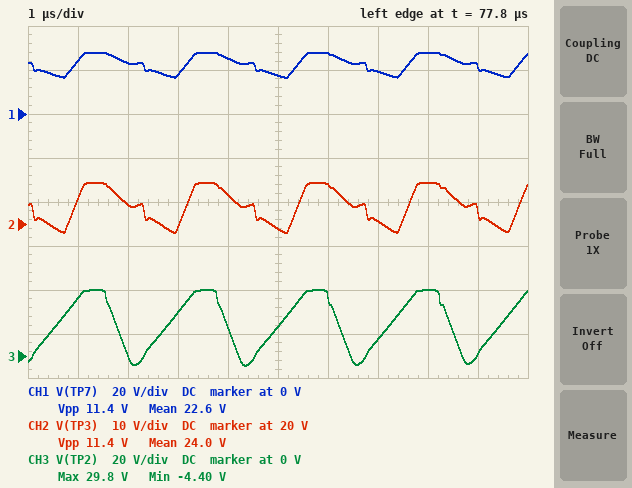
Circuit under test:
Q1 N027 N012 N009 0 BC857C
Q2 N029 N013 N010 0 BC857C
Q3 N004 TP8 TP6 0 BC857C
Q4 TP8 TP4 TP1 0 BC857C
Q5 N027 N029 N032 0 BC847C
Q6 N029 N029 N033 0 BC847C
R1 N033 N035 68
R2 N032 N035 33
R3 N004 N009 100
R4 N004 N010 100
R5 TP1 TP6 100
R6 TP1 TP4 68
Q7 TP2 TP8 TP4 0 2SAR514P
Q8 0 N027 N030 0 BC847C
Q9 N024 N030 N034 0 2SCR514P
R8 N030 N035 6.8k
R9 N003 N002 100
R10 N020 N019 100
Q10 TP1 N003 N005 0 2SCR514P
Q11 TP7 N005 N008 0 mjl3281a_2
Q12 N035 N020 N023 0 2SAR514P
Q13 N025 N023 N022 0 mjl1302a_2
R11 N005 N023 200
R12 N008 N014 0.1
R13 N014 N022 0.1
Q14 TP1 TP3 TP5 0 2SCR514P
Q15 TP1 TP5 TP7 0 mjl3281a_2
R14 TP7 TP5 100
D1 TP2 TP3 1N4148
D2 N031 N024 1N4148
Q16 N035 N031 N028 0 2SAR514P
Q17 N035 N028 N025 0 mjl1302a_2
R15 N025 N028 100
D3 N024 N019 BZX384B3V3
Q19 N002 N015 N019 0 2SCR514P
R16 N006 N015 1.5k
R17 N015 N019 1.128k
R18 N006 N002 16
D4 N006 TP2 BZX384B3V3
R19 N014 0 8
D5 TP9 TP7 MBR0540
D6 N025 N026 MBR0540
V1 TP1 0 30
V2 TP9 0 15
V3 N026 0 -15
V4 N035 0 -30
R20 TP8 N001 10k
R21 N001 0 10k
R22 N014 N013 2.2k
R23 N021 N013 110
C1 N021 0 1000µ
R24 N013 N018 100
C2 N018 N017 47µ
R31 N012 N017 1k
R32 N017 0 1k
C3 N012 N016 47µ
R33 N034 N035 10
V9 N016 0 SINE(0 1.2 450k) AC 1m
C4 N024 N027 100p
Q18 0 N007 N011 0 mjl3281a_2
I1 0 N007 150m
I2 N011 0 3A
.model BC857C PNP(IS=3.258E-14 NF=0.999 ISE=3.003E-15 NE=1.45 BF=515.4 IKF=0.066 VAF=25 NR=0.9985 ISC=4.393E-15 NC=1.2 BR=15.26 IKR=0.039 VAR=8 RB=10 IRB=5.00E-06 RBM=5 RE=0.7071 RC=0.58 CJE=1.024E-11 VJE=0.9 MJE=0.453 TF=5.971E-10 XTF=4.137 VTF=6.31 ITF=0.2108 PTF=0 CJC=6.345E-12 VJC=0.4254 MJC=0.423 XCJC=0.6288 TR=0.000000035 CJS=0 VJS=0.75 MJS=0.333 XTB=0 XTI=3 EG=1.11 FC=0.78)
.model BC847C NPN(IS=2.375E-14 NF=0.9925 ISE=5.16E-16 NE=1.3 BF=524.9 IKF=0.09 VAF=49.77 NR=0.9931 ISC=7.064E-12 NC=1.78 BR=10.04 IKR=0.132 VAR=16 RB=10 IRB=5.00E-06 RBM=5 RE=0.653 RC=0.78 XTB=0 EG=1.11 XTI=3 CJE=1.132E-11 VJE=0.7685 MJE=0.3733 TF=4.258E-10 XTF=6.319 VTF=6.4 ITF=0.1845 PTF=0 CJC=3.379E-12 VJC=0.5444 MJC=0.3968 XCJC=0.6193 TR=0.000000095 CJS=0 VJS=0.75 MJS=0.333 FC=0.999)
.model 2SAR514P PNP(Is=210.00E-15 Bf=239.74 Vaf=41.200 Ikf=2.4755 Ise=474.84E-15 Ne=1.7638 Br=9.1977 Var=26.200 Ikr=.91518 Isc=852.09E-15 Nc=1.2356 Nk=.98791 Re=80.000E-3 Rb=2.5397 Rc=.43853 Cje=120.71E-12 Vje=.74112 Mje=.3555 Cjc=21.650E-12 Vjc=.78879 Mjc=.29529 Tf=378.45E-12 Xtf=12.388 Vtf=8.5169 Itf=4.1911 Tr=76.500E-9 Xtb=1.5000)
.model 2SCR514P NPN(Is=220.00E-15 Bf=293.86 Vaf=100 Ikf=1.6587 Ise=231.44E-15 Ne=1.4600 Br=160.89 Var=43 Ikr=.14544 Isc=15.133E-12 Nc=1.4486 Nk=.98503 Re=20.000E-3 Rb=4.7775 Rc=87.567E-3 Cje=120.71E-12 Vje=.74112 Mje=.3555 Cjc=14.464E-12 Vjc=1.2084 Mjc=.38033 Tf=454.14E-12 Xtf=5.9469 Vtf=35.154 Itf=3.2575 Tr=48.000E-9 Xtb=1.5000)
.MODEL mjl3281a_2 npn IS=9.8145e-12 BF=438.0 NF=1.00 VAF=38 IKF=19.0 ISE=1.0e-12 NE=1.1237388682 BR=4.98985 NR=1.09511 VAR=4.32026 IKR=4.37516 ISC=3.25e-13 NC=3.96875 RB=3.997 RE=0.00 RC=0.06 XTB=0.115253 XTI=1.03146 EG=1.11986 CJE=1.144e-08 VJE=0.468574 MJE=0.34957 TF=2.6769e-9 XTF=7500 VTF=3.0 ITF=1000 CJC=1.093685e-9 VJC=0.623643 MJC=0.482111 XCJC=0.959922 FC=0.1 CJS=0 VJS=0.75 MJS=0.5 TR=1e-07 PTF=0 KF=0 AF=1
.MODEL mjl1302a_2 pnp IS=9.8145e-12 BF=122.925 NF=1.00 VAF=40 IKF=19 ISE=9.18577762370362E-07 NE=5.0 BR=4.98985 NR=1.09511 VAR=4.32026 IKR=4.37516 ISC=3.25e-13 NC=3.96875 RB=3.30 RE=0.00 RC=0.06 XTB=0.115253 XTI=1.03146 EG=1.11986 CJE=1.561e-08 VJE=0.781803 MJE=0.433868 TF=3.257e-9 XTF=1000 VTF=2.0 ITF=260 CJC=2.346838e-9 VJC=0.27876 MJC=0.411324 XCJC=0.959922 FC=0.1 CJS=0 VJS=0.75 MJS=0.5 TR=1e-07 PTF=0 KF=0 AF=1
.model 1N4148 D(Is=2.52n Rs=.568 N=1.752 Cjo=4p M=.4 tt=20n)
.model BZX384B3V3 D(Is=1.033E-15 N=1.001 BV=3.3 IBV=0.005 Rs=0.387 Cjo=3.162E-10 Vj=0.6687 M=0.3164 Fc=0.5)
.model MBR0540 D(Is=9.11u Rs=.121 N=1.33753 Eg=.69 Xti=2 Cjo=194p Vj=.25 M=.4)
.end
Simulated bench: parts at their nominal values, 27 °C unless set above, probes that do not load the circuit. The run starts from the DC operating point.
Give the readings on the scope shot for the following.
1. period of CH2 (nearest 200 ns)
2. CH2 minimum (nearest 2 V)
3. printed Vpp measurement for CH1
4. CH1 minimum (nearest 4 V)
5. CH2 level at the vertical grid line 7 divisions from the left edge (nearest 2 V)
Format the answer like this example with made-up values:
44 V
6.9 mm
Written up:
2.2 µs
18 V
11.4 V
16 V
20 V
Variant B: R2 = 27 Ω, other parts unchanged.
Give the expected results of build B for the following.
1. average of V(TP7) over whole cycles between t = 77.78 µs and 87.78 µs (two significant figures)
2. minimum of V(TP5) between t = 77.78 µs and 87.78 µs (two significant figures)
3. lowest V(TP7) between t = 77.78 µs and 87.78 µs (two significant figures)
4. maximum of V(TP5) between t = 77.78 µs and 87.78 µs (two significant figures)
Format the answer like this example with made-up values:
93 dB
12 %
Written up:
24 V
18 V
17 V
29 V
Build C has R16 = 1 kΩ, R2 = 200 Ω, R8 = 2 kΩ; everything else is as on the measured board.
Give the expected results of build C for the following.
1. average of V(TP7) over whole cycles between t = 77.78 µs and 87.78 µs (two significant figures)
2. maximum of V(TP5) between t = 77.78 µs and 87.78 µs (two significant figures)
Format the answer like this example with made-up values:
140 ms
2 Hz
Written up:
15 V
19 V
